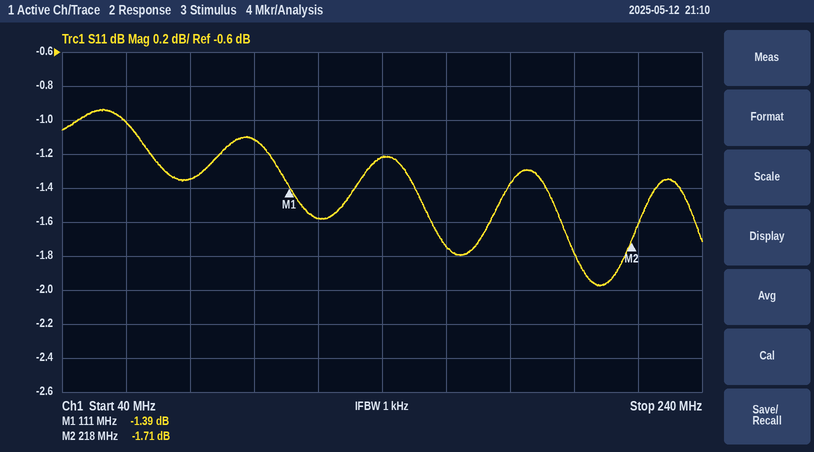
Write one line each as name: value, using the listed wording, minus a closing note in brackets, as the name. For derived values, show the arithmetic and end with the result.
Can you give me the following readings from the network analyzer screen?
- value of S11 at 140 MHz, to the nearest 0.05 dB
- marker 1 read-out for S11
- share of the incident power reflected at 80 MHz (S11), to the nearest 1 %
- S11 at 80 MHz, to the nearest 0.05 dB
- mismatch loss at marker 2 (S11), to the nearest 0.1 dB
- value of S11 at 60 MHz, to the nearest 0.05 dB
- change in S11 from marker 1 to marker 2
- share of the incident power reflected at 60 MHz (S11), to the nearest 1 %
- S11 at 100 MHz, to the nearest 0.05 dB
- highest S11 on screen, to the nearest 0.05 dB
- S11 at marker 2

value of S11 at 140 MHz, to the nearest 0.05 dB: -1.20 dB
marker 1 read-out for S11: -1.39 dB
share of the incident power reflected at 80 MHz (S11), to the nearest 1 %: 10^(-1.35/10) ≈ 73 %
S11 at 80 MHz, to the nearest 0.05 dB: -1.35 dB
mismatch loss at marker 2 (S11), to the nearest 0.1 dB: −10 log10(1 − 10^(-1.71/10)) ≈ 4.9 dB
value of S11 at 60 MHz, to the nearest 0.05 dB: -1.00 dB
change in S11 from marker 1 to marker 2: -1.71 − (-1.39) = -0.32 dB
share of the incident power reflected at 60 MHz (S11), to the nearest 1 %: 10^(-1/10) ≈ 79 %
S11 at 100 MHz, to the nearest 0.05 dB: -1.10 dB
highest S11 on screen, to the nearest 0.05 dB: -0.95 dB
S11 at marker 2: -1.71 dB
